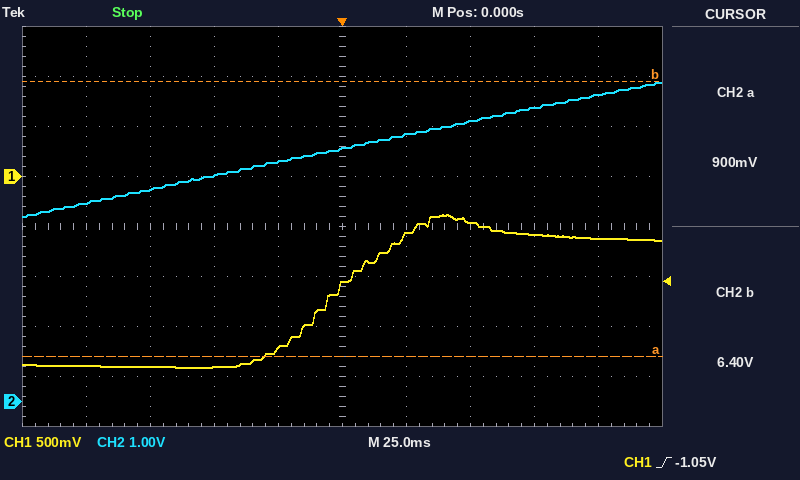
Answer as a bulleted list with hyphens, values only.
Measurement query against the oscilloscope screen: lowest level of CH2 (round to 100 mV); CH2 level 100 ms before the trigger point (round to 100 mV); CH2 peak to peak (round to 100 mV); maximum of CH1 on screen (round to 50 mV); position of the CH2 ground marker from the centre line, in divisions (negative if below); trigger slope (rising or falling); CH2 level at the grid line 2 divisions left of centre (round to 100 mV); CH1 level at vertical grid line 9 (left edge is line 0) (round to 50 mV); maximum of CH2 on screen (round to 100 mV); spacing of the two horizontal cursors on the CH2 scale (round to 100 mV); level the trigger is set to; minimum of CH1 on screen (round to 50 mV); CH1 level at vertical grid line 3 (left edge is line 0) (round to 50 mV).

- 3.7 V
- 4.0 V
- 2.7 V
- -400 mV
- -3.5 div
- rising
- 4.5 V
- -600 mV
- 6.4 V
- 5.5 V
- -1.05 V
- -1.90 V
- -1.90 V
